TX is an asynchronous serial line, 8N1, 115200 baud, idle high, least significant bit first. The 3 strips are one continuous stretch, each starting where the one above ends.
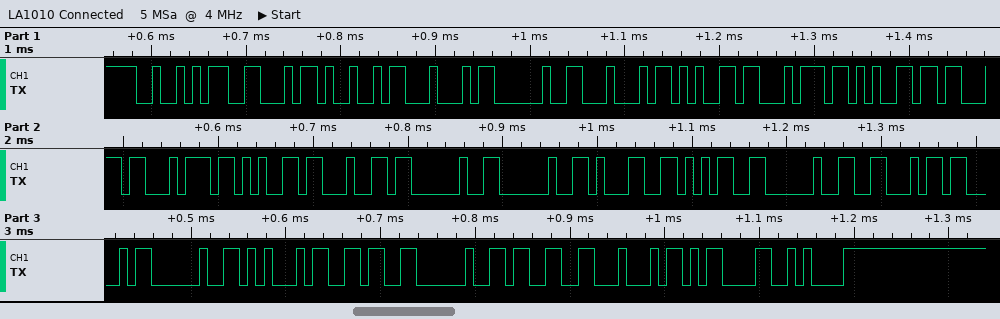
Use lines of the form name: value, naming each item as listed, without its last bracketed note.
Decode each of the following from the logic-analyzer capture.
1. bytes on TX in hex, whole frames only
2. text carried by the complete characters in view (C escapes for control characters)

bytes on TX in hex, whole frames only: 0x52 0x46 0x49 0x44 0x20 0x44 0x65 0x74 0x65 0x63 0x74 0x65 0x64 0x20 0x20 0x31 0x35 0x20 0x46 0x43 0x20 0x45 0x36 0x20 0x33 0x44 0x0D 0x0A
text carried by the complete characters in view: "RFID Detected  15 FC E6 3D\r\n"
